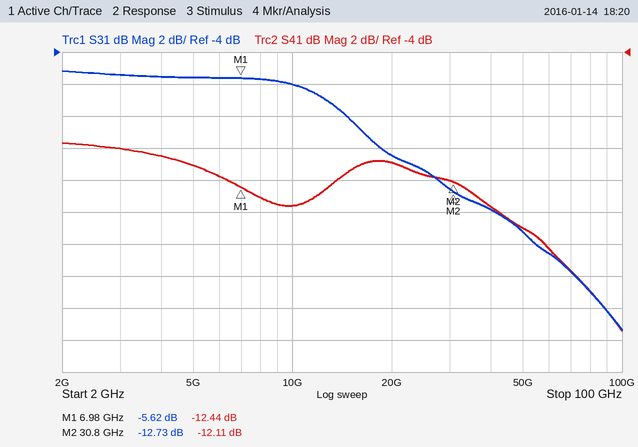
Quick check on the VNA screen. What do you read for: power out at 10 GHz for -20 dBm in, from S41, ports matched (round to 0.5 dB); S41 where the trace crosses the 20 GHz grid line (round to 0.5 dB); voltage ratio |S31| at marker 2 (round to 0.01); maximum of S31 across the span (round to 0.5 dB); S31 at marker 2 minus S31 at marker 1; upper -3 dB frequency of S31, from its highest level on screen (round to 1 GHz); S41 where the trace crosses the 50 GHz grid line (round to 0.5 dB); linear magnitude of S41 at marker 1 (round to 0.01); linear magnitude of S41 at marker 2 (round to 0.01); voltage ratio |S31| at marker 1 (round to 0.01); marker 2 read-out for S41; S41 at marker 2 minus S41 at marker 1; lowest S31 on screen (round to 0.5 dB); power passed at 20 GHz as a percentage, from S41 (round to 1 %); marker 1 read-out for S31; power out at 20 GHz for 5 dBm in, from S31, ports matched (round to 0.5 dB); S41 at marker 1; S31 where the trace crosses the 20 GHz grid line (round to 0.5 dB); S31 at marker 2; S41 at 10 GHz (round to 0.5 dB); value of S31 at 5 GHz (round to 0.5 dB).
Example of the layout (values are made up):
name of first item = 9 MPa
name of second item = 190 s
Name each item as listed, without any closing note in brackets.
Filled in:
power out at 10 GHz for -20 dBm in, from S41, ports matched = -33.5 dBm
S41 where the trace crosses the 20 GHz grid line = -11.0 dB
voltage ratio |S31| at marker 2 = 0.23
maximum of S31 across the span = -5.0 dB
S31 at marker 2 minus S31 at marker 1 = -7.11 dB
upper -3 dB frequency of S31, from its highest level on screen = 15 GHz
S41 where the trace crosses the 50 GHz grid line = -15.0 dB
linear magnitude of S41 at marker 1 = 0.24
linear magnitude of S41 at marker 2 = 0.25
voltage ratio |S31| at marker 1 = 0.52
marker 2 read-out for S41 = -12.11 dB
S41 at marker 2 minus S41 at marker 1 = 0.33 dB
lowest S31 on screen = -21.5 dB
power passed at 20 GHz as a percentage, from S41 = 8 %
marker 1 read-out for S31 = -5.62 dB
power out at 20 GHz for 5 dBm in, from S31, ports matched = -5.5 dBm
S41 at marker 1 = -12.44 dB
S31 where the trace crosses the 20 GHz grid line = -10.5 dB
S31 at marker 2 = -12.73 dB
S41 at 10 GHz = -13.5 dB
value of S31 at 5 GHz = -5.5 dB
